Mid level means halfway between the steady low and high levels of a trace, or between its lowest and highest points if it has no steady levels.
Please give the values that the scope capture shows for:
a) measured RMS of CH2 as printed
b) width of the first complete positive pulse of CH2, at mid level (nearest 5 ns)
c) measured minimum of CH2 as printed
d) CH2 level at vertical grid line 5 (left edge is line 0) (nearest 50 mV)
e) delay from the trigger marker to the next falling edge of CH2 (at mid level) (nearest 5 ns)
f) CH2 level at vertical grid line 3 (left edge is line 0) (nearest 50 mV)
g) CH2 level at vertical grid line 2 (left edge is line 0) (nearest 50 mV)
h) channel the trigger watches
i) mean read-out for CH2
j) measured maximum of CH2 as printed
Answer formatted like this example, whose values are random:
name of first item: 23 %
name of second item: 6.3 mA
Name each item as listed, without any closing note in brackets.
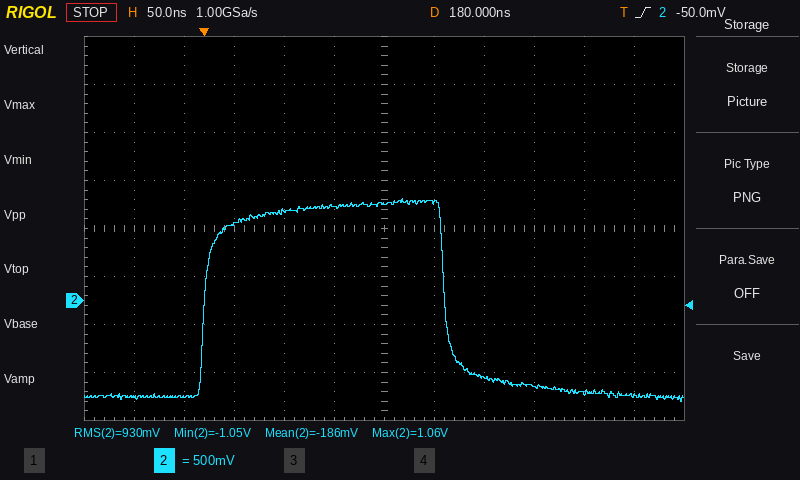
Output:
measured RMS of CH2 as printed: 930 mV
width of the first complete positive pulse of CH2, at mid level: 240 ns
measured minimum of CH2 as printed: -1.05 V
CH2 level at vertical grid line 5 (left edge is line 0): 1.00 V
delay from the trigger marker to the next falling edge of CH2 (at mid level): 240 ns
CH2 level at vertical grid line 3 (left edge is line 0): 800 mV
CH2 level at vertical grid line 2 (left edge is line 0): -1.00 V
channel the trigger watches: CH2
mean read-out for CH2: -186 mV
measured maximum of CH2 as printed: 1.06 V
